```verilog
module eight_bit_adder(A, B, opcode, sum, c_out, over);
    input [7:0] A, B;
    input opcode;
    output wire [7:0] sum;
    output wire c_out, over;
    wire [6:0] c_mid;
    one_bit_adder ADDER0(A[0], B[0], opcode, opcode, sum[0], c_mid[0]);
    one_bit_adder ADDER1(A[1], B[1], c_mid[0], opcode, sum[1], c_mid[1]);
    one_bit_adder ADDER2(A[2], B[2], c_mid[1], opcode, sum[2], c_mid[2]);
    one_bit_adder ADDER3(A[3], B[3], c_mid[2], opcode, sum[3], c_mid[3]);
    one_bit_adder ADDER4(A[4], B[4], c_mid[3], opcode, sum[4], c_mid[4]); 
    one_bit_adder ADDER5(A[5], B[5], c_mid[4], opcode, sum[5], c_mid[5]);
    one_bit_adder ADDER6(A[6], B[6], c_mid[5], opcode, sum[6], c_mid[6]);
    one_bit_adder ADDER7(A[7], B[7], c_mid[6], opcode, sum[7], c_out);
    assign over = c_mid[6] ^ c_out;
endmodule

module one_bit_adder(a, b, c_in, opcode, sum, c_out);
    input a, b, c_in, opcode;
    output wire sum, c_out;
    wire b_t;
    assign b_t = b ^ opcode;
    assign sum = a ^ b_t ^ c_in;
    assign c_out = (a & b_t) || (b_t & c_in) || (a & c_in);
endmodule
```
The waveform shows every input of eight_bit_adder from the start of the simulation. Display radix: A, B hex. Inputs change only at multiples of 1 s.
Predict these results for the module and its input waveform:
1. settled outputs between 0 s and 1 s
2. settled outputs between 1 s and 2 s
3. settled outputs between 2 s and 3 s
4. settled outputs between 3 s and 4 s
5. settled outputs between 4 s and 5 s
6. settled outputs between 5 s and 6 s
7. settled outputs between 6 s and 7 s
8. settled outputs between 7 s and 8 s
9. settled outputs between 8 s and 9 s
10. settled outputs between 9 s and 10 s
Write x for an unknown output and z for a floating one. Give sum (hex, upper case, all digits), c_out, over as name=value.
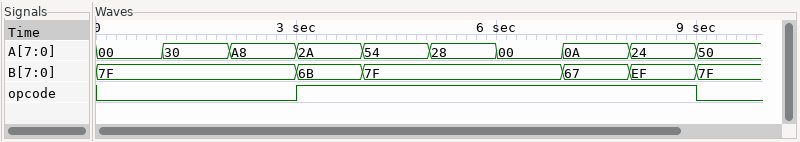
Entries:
sum=7F, c_out=0, over=0
sum=AF, c_out=0, over=1
sum=27, c_out=1, over=0
sum=BF, c_out=0, over=0
sum=D5, c_out=0, over=0
sum=A9, c_out=0, over=0
sum=81, c_out=0, over=0
sum=A3, c_out=0, over=0
sum=35, c_out=0, over=0
sum=CF, c_out=0, over=1
